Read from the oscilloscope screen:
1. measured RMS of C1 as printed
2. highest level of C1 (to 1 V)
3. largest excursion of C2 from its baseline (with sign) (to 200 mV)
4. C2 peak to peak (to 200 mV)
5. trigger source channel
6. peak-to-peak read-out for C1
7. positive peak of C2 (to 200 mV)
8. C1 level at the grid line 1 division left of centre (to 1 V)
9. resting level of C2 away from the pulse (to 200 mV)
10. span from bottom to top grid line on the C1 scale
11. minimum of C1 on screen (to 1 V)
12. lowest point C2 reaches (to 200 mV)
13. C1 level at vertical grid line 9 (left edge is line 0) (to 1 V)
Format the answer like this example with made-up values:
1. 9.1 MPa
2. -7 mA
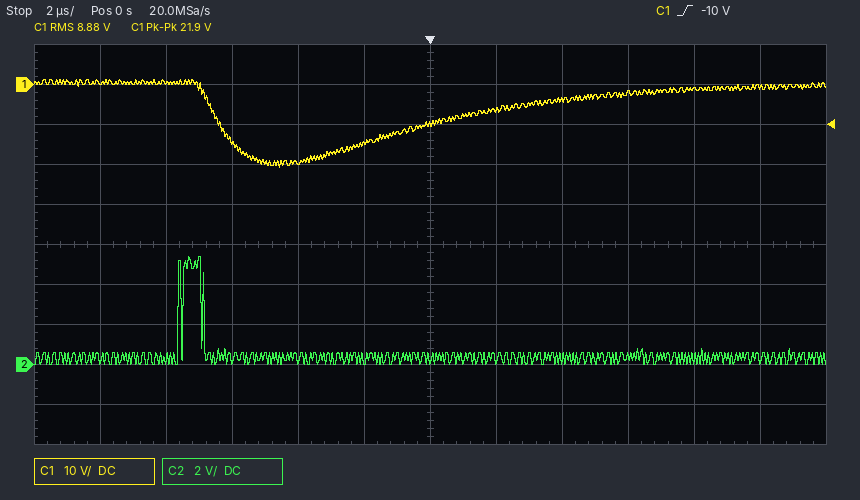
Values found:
1. 8.88 V
2. 1 V
3. +5.0 V
4. 5.4 V
5. C1
6. 21.9 V
7. 5.4 V
8. -15 V
9. 400 mV
10. 100 V
11. -21 V
12. 0.0 V
13. -2 V
